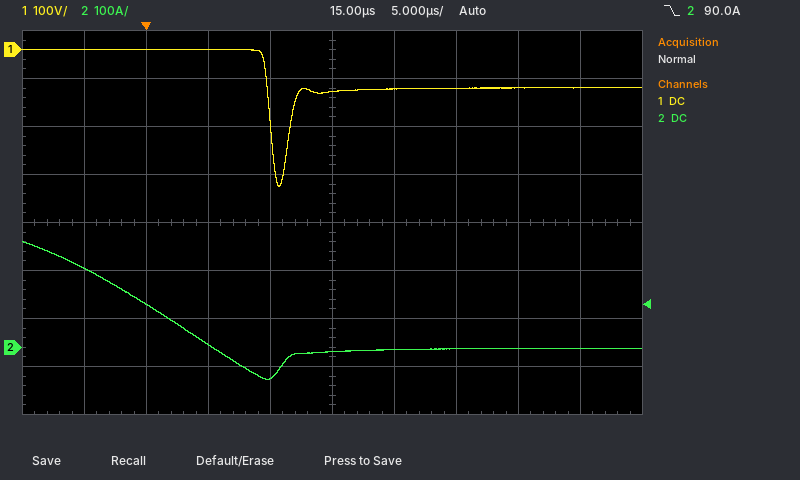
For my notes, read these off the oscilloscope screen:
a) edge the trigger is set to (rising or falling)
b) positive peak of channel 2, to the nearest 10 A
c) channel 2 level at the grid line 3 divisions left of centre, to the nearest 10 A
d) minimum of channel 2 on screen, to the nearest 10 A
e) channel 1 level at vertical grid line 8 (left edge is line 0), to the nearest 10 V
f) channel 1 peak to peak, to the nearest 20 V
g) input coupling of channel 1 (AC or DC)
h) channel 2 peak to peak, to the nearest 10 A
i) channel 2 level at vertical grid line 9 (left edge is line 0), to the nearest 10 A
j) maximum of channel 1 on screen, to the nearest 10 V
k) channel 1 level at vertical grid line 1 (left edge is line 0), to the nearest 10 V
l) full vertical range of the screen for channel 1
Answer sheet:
falling
220 A
90 A
-70 A
-80 V
280 V
DC
290 A
0 A
0 V
0 V
800 V
